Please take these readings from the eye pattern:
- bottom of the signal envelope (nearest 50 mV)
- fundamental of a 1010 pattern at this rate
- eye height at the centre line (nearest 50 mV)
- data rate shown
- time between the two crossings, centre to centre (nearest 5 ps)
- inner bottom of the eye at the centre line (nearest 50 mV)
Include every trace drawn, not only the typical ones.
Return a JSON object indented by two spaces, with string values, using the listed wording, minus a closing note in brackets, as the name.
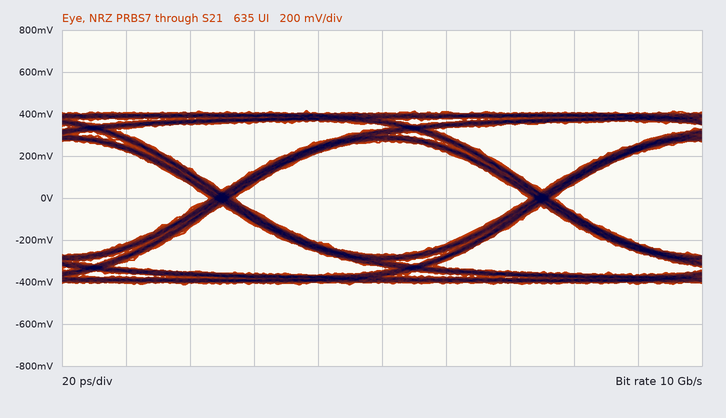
{
  "bottom of the signal envelope": "-400 mV",
  "fundamental of a 1010 pattern at this rate": "5 GHz",
  "eye height at the centre line": "550 mV",
  "data rate shown": "10 Gb/s",
  "time between the two crossings, centre to centre": "100 ps",
  "inner bottom of the eye at the centre line": "-250 mV"
}
